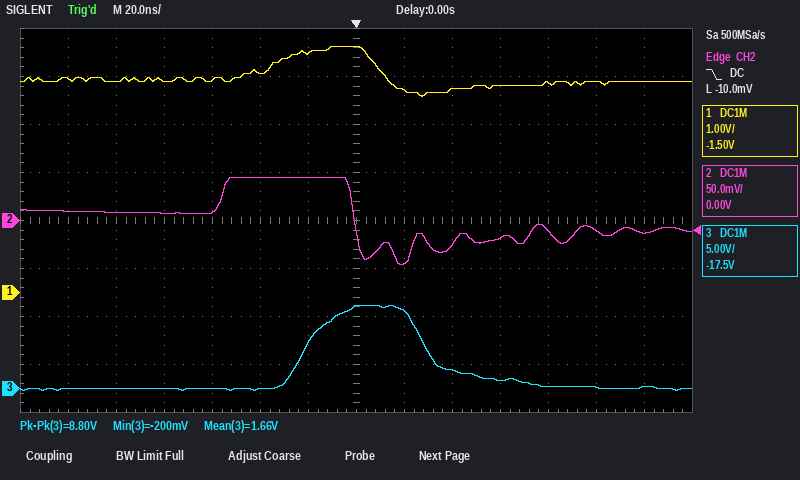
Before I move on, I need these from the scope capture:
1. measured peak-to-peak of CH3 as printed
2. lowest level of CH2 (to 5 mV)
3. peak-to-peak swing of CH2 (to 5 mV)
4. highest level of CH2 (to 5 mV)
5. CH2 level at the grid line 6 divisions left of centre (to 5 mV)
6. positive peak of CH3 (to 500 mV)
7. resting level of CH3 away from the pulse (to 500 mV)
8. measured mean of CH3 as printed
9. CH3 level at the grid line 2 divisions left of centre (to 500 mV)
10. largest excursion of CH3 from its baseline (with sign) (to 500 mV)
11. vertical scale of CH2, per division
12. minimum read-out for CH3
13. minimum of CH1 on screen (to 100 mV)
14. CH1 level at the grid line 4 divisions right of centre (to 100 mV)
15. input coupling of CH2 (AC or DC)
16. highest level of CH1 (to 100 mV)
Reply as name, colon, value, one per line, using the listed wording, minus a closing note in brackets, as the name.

measured peak-to-peak of CH3 as printed: 8.80 V
lowest level of CH2: -45 mV
peak-to-peak swing of CH2: 90 mV
highest level of CH2: 45 mV
CH2 level at the grid line 6 divisions left of centre: 10 mV
positive peak of CH3: 8.5 V
resting level of CH3 away from the pulse: 0.0 V
measured mean of CH3 as printed: 1.66 V
CH3 level at the grid line 2 divisions left of centre: 0.0 V
largest excursion of CH3 from its baseline (with sign): +8.5 V
vertical scale of CH2, per division: 50 mV
minimum read-out for CH3: -200 mV
minimum of CH1 on screen: 4.1 V
CH1 level at the grid line 4 divisions right of centre: 4.4 V
input coupling of CH2: DC
highest level of CH1: 5.1 V
